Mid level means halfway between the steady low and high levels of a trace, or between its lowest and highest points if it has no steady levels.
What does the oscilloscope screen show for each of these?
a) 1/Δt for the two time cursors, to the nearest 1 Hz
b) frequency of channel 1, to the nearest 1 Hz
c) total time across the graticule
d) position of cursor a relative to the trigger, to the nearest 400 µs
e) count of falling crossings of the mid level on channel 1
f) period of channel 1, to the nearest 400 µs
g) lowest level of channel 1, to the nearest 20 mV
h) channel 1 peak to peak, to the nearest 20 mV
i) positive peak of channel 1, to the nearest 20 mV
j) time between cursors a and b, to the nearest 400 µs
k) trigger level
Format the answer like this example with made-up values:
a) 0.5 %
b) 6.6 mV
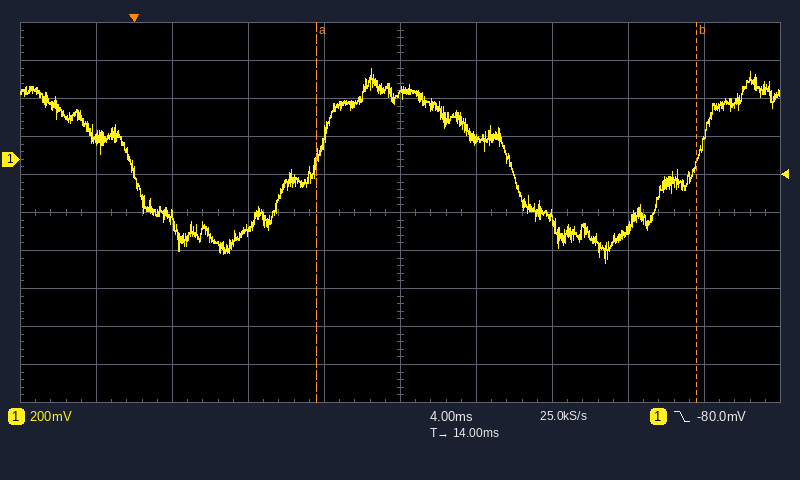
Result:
a) 50 Hz
b) 50 Hz
c) 40 ms
d) +9.6 ms
e) 2
f) 20.0 ms
g) -540 mV
h) 1.02 V
i) 480 mV
j) 20.0 ms
k) -80.0 mV
